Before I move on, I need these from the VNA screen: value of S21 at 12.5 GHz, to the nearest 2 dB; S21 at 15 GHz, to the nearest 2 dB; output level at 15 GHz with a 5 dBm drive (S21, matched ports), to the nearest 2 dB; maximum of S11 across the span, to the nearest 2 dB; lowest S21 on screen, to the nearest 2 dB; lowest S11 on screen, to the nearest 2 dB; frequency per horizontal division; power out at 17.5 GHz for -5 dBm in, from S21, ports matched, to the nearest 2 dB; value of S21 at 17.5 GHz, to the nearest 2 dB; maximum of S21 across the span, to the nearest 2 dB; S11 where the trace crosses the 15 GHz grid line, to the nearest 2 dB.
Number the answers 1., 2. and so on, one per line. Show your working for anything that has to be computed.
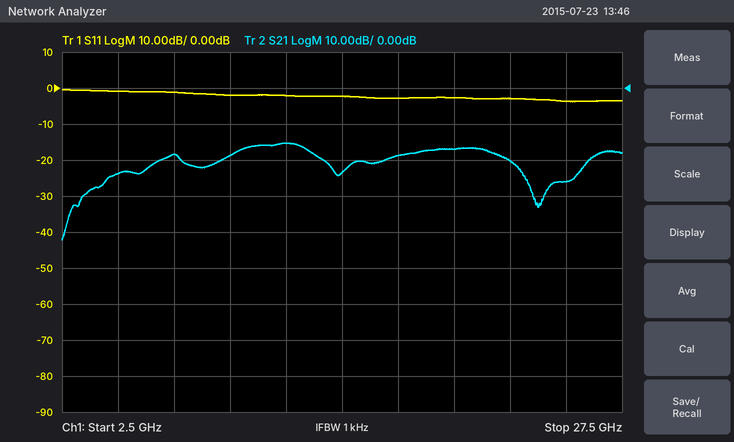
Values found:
1. -16 dB
2. -24 dB
3. 5 dBm + (-24 dB) = -18 dBm
4. 0 dB
5. -42 dB
6. -4 dB
7. 2.5 GHz
8. -5 dBm + (-18 dB) = -24 dBm
9. -18 dB
10. -16 dB
11. -2 dB
